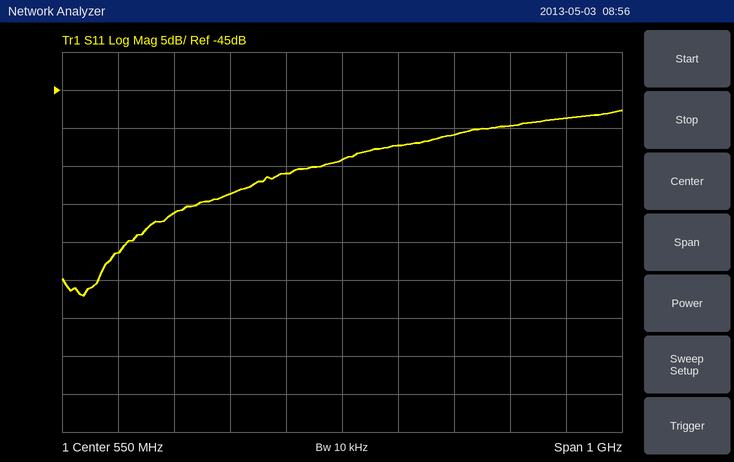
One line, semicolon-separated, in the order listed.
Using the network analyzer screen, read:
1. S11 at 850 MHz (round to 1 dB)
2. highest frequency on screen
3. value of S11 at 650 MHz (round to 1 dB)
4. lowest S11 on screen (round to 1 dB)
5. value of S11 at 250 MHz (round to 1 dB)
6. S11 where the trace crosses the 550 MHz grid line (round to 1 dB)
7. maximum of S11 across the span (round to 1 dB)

-50 dB; 1.05 GHz; -52 dB; -72 dB; -61 dB; -54 dB; -48 dB
